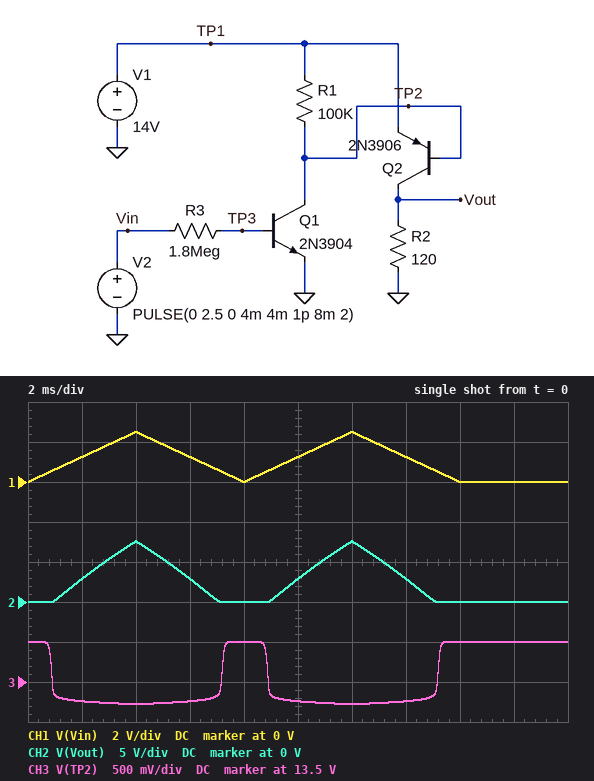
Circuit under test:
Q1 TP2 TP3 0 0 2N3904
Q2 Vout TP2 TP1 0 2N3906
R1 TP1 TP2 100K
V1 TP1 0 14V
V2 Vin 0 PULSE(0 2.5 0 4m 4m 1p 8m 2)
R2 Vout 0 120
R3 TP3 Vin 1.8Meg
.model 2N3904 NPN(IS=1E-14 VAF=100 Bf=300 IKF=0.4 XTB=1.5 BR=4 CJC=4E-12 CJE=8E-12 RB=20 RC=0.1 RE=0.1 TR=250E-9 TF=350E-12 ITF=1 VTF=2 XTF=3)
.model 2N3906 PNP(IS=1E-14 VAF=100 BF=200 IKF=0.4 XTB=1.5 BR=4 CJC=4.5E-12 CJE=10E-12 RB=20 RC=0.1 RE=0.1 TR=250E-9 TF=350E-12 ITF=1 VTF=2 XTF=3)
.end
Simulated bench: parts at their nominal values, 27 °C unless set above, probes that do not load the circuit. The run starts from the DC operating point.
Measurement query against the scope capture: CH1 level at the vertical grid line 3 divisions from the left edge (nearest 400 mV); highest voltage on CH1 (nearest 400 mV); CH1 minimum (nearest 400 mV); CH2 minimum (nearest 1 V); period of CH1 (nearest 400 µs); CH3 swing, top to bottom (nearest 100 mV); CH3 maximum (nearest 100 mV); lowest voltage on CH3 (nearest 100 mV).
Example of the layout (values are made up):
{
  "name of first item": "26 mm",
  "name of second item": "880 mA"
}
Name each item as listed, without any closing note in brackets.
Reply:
{
  "CH1 level at the vertical grid line 3 divisions from the left edge": "1.2 V",
  "highest voltage on CH1": "2.4 V",
  "CH1 minimum": "0 V",
  "CH2 minimum": "0 V",
  "period of CH1": "8.0 ms",
  "CH3 swing, top to bottom": "800 mV",
  "CH3 maximum": "14.0 V",
  "lowest voltage on CH3": "13.2 V"
}
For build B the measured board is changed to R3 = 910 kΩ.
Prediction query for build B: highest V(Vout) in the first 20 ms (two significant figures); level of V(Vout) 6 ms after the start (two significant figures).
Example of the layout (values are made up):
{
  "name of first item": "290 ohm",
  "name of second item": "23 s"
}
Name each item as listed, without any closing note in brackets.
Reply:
{
  "highest V(Vout) in the first 20 ms": "13 V",
  "level of V(Vout) 6 ms after the start": "5.4 V"
}
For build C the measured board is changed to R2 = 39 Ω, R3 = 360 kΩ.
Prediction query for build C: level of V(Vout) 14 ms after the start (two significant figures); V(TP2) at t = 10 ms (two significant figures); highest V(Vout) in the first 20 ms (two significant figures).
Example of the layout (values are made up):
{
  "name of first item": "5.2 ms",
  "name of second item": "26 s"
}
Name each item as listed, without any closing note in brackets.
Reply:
{
  "level of V(Vout) 14 ms after the start": "3.9 V",
  "V(TP2) at t = 10 ms": "13 V",
  "highest V(Vout) in the first 20 ms": "8.9 V"
}
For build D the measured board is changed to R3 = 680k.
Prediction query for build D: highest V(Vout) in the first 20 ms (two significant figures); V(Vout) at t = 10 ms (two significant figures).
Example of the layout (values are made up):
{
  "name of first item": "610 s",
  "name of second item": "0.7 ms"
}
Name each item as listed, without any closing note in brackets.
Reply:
{
  "highest V(Vout) in the first 20 ms": "14 V",
  "V(Vout) at t = 10 ms": "6.8 V"
}
